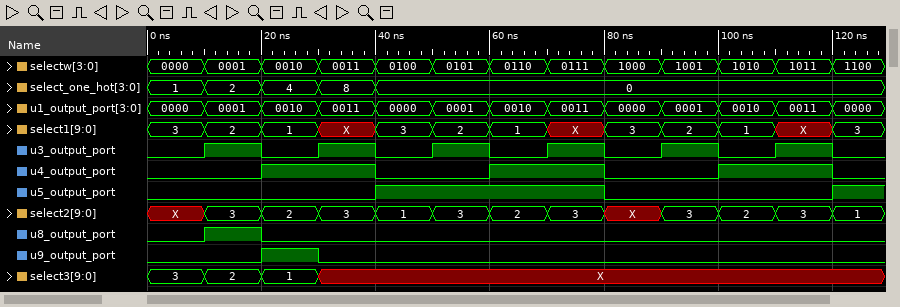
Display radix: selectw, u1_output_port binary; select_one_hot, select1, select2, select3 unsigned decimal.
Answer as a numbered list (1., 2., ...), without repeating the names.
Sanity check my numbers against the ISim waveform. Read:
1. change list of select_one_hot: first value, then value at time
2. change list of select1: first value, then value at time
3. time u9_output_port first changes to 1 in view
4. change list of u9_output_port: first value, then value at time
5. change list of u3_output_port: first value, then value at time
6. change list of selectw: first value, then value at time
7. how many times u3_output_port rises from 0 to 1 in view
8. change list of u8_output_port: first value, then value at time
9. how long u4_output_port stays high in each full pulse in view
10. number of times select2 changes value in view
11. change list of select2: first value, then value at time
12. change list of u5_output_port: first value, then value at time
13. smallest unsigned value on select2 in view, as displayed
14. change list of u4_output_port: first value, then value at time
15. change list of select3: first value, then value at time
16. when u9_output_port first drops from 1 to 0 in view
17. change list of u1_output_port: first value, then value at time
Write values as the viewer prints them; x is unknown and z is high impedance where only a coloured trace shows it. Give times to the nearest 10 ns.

1. 1, 2 at 10 ns, 4 at 20 ns, 8 at 30 ns, 0 at 40 ns
2. 3, 2 at 10 ns, 1 at 20 ns, X at 30 ns, 3 at 40 ns, 2 at 50 ns, 1 at 60 ns, X at 70 ns, 3 at 80 ns, 2 at 90 ns, 1 at 100 ns, X at 110 ns, 3 at 120 ns
3. 20 ns
4. 0, 1 at 20 ns, 0 at 30 ns
5. 0, 1 at 10 ns, 0 at 20 ns, 1 at 30 ns, 0 at 40 ns, 1 at 50 ns, 0 at 60 ns, 1 at 70 ns, 0 at 80 ns, 1 at 90 ns, 0 at 100 ns, 1 at 110 ns, 0 at 120 ns
6. 0000, 0001 at 10 ns, 0010 at 20 ns, 0011 at 30 ns, 0100 at 40 ns, 0101 at 50 ns, 0110 at 60 ns, 0111 at 70 ns, 1000 at 80 ns, 1001 at 90 ns, 1010 at 100 ns, 1011 at 110 ns, 1100 at 120 ns
7. 6
8. 0, 1 at 10 ns, 0 at 20 ns
9. 20 ns, 20 ns, 20 ns
10. 12
11. X, 3 at 10 ns, 2 at 20 ns, 3 at 30 ns, 1 at 40 ns, 3 at 50 ns, 2 at 60 ns, 3 at 70 ns, X at 80 ns, 3 at 90 ns, 2 at 100 ns, 3 at 110 ns, 1 at 120 ns
12. 0, 1 at 40 ns, 0 at 80 ns, 1 at 120 ns
13. 1
14. 0, 1 at 20 ns, 0 at 40 ns, 1 at 60 ns, 0 at 80 ns, 1 at 100 ns, 0 at 120 ns
15. 3, 2 at 10 ns, 1 at 20 ns, X at 30 ns
16. 30 ns
17. 0000, 0001 at 10 ns, 0010 at 20 ns, 0011 at 30 ns, 0000 at 40 ns, 0001 at 50 ns, 0010 at 60 ns, 0011 at 70 ns, 0000 at 80 ns, 0001 at 90 ns, 0010 at 100 ns, 0011 at 110 ns, 0000 at 120 ns
